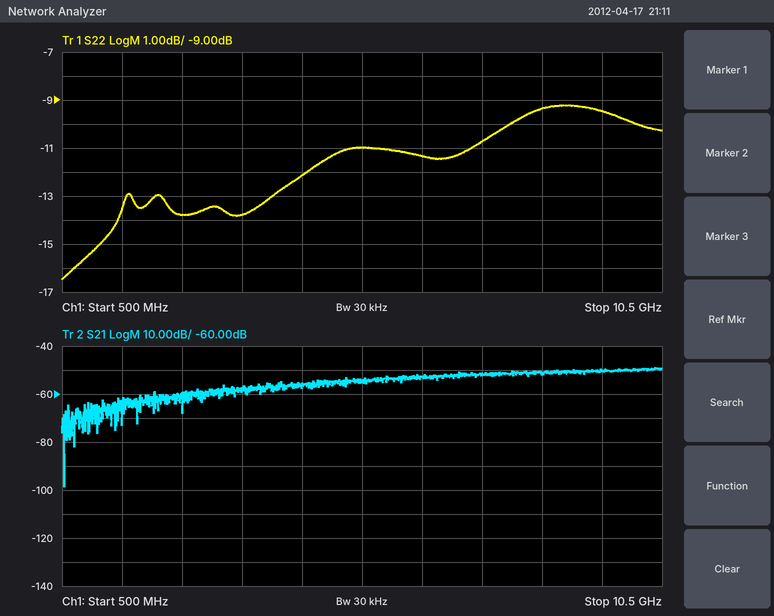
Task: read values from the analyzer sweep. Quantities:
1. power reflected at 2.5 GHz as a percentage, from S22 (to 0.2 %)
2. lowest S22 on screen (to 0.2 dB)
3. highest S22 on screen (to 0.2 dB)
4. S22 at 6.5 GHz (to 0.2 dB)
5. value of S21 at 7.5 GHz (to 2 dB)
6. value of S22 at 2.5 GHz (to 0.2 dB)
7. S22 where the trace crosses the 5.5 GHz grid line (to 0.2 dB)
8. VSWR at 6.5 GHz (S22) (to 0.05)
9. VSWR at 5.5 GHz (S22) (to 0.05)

4.2 %
-16.4 dB
-9.2 dB
-11.4 dB
-52 dB
-13.8 dB
-11.0 dB
1.75
1.80
